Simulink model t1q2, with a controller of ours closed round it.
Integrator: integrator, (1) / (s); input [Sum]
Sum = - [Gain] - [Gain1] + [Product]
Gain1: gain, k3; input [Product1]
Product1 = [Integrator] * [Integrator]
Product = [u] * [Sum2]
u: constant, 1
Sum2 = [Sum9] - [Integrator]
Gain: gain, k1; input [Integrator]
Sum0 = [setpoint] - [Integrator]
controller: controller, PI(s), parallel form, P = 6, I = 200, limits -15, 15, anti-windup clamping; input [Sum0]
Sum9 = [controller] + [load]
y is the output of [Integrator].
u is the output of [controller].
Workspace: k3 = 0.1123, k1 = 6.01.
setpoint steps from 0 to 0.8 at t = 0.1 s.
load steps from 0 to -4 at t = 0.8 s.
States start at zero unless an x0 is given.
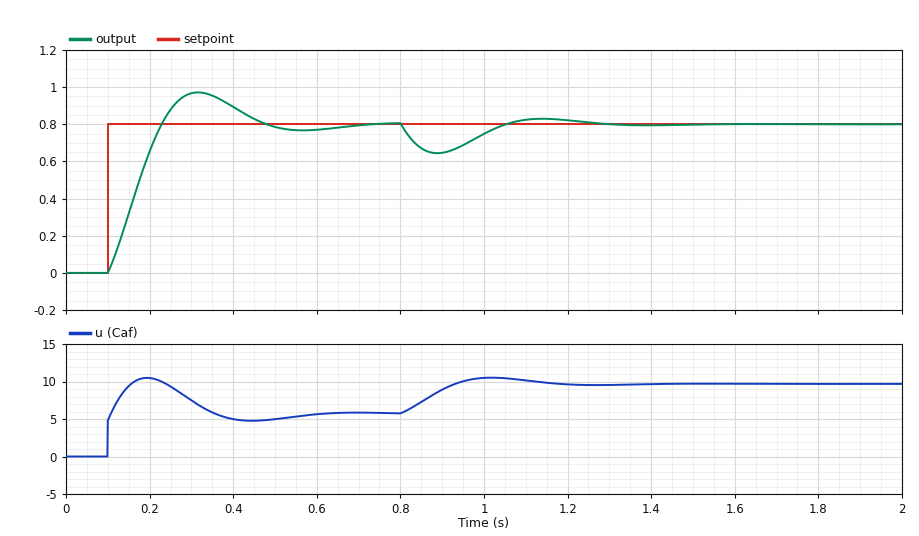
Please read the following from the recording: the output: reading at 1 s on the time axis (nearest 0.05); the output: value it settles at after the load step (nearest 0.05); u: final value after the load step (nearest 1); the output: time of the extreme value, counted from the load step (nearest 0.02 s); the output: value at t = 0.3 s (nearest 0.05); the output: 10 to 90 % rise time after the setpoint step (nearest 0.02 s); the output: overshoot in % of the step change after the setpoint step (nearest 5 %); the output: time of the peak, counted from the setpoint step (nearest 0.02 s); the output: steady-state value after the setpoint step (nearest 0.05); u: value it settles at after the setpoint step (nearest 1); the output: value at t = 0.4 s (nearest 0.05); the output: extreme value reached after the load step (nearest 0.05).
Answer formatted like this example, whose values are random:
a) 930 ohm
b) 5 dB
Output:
a) 0.75
b) 0.80
c) 10
d) 0.08 s
e) 0.95
f) 0.10 s
g) 20 %
h) 0.22 s
i) 0.80
j) 6
k) 0.90
l) 0.65
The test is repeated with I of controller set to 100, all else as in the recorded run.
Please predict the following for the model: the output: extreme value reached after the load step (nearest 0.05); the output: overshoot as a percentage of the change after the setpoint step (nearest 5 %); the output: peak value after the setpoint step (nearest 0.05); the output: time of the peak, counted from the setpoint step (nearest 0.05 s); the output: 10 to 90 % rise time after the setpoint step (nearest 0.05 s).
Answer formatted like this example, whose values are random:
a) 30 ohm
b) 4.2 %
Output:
a) 0.60
b) 10 %
c) 0.85
d) 0.35 s
e) 0.15 s
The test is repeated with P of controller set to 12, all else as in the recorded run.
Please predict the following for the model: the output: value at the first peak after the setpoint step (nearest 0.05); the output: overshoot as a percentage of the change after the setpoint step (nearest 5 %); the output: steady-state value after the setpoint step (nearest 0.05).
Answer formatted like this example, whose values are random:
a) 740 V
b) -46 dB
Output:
a) 0.90
b) 10 %
c) 0.80
